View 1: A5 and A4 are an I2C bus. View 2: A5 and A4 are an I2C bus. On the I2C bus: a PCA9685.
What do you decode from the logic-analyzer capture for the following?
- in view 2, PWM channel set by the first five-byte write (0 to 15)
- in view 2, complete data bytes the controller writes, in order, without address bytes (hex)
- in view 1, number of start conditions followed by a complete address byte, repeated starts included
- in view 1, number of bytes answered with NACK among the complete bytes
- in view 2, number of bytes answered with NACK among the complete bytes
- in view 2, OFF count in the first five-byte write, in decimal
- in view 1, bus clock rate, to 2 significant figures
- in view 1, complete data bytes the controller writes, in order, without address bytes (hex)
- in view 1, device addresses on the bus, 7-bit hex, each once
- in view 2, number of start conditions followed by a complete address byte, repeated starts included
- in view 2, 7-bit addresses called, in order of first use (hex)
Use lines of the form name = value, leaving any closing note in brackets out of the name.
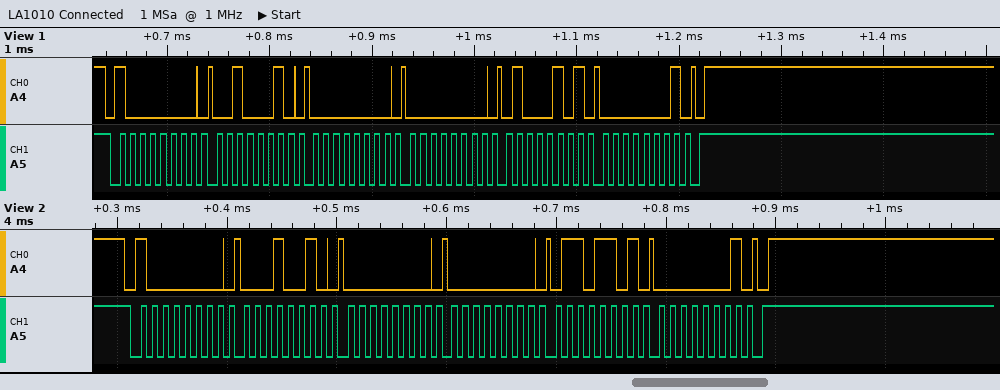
in view 2, PWM channel set by the first five-byte write = 3
in view 2, complete data bytes the controller writes, in order, without address bytes = 12 00 00 6D 01
in view 1, number of start conditions followed by a complete address byte, repeated starts included = 1
in view 1, number of bytes answered with NACK among the complete bytes = 0
in view 2, number of bytes answered with NACK among the complete bytes = 0
in view 2, OFF count in the first five-byte write, in decimal = 365
in view 1, bus clock rate, to 2 significant figures = 100 kHz
in view 1, complete data bytes the controller writes, in order, without address bytes = 22 00 00 45 01
in view 1, device addresses on the bus, 7-bit hex, each once = 0x40
in view 2, number of start conditions followed by a complete address byte, repeated starts included = 1
in view 2, 7-bit addresses called, in order of first use = 0x40
